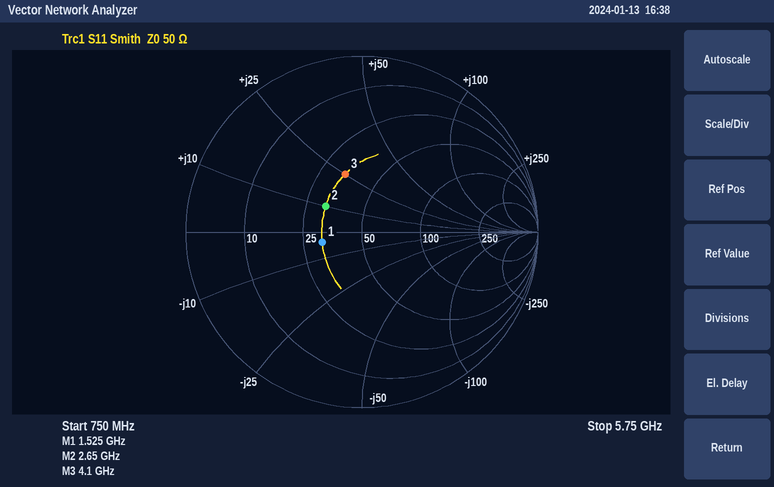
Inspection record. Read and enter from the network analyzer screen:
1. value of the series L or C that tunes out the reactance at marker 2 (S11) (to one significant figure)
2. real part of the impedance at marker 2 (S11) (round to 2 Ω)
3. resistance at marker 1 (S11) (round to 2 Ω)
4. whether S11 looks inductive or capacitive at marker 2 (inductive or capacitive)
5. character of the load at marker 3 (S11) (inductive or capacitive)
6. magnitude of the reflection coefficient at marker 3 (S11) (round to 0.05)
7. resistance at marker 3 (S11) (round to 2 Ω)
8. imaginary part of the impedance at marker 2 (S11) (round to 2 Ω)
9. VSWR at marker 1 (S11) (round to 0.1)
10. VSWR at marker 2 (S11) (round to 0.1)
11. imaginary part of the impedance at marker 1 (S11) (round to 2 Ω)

6 pF
32 Ω
32 Ω
inductive
inductive
0.35
34 Ω
+10 Ω
1.6
1.7
-4 Ω
